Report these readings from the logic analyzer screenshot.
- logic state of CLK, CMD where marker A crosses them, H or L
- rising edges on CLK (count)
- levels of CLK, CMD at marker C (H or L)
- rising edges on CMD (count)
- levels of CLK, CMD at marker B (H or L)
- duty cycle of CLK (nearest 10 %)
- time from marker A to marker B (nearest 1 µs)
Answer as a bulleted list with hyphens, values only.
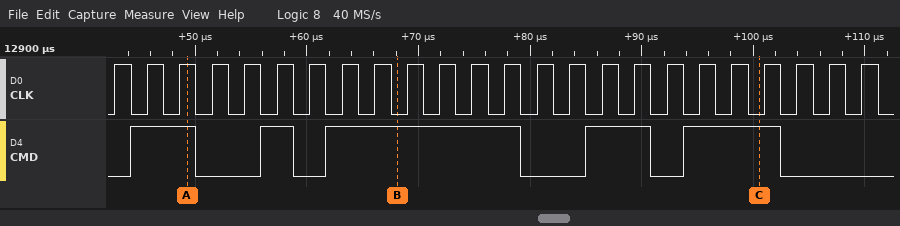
- CLK=H, CMD=H
- 24
- CLK=L, CMD=H
- 5
- CLK=L, CMD=H
- 50 %
- 19 µs
